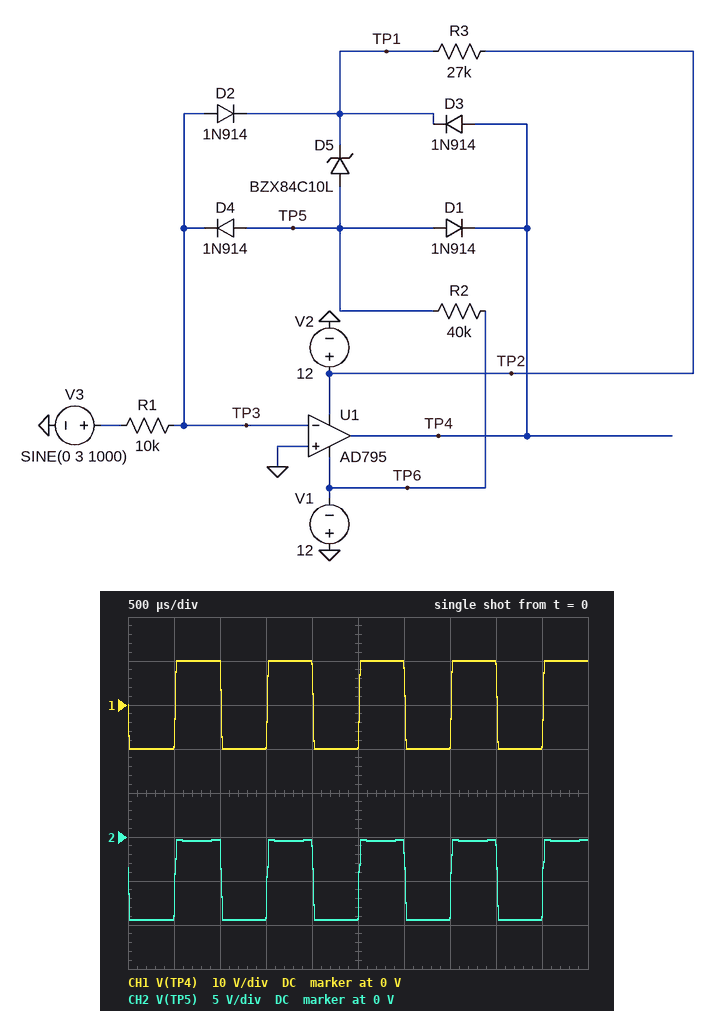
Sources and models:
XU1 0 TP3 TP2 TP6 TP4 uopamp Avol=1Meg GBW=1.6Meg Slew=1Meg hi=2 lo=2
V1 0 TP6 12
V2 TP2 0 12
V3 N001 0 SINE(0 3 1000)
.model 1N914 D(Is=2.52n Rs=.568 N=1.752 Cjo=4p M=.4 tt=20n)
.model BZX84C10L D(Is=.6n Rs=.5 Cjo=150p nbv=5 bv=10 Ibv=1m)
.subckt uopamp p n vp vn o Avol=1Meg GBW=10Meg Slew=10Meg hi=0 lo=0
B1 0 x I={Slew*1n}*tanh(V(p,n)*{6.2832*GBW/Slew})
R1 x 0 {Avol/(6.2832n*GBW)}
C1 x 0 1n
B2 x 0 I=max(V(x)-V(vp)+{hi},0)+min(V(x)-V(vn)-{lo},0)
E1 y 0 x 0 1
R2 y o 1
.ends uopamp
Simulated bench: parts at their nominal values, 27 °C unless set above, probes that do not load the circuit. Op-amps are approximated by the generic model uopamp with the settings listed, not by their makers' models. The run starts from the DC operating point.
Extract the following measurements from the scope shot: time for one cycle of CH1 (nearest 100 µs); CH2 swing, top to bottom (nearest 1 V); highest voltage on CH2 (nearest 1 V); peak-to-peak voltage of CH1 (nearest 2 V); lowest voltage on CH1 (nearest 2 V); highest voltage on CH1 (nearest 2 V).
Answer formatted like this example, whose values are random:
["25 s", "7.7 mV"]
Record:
["1.0 ms", "9 V", "0 V", "20 V", "-10 V", "10 V"]
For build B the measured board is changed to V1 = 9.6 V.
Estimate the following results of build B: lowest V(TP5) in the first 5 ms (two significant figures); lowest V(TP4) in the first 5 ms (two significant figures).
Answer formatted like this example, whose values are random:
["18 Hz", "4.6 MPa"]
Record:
["-7.1 V", "-7.6 V"]
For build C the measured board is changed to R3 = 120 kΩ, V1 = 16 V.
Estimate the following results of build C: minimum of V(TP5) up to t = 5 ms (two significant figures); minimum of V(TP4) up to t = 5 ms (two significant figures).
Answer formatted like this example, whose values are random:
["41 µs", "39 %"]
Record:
["-10 V", "-11 V"]
